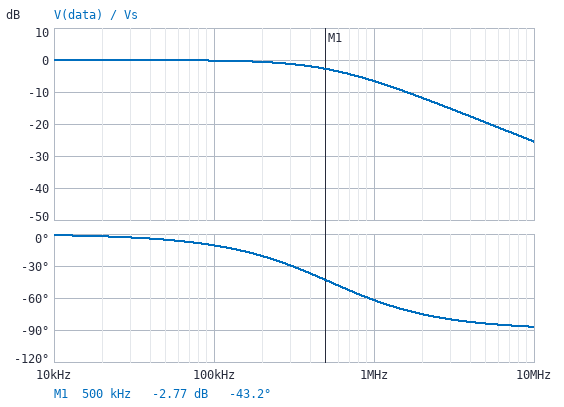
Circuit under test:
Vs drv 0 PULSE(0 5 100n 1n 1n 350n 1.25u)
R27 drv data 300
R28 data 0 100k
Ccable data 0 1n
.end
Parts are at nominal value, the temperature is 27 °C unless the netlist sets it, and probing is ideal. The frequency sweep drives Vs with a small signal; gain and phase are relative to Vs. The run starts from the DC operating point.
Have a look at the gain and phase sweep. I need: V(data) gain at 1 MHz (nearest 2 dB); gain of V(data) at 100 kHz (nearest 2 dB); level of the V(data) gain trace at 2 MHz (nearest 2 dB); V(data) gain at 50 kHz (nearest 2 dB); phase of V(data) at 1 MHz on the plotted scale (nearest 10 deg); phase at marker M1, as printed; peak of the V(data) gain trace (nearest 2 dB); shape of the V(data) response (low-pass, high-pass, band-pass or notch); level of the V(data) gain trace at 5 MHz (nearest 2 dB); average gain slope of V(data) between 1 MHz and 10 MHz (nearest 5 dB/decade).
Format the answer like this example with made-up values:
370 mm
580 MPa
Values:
-6 dB
0 dB
-12 dB
0 dB
-60 deg
-43.2 deg
0 dB
low-pass
-20 dB
-20 dB/decade
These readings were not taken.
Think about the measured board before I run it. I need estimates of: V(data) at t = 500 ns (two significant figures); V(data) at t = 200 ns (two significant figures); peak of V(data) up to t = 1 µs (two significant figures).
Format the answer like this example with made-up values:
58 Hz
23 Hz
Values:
2.9 V
1.4 V
3.4 V
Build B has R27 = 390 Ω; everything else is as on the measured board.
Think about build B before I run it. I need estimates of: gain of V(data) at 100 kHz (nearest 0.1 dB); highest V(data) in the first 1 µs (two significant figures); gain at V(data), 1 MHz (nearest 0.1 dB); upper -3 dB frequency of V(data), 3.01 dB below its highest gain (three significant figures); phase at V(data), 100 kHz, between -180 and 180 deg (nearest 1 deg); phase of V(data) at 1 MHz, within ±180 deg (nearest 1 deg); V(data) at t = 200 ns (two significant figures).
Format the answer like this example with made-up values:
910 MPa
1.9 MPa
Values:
-0.3 dB
3.0 V
-8.5 dB
410 kHz
-14 deg
-68 deg
1.1 V
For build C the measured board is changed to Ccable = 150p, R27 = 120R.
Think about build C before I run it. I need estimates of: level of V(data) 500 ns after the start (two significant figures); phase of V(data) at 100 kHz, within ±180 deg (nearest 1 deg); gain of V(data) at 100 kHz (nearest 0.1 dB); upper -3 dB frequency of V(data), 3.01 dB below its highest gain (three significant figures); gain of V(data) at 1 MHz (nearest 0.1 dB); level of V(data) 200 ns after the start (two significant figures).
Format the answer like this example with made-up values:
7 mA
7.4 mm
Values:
340 mV
-1 deg
0 dB
8.85 MHz
-0.1 dB
5.0 V
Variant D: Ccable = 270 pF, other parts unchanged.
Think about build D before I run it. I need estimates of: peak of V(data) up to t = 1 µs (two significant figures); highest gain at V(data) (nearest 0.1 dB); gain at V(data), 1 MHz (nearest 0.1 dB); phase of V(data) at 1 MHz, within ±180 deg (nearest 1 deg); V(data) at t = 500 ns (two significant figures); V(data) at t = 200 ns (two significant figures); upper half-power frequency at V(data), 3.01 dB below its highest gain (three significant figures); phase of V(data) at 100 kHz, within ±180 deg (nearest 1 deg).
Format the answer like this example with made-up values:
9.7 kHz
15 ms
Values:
4.9 V
0 dB
-1.0 dB
-27 deg
2.7 V
3.5 V
1.97 MHz
-3 deg
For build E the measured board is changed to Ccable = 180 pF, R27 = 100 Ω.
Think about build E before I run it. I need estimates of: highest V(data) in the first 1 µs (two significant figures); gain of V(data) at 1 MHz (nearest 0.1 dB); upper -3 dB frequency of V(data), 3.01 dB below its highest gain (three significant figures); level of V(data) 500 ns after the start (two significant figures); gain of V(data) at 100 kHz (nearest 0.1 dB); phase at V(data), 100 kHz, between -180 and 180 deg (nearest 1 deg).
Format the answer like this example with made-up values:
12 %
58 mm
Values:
5.0 V
-0.1 dB
8.85 MHz
340 mV
0 dB
-1 deg
